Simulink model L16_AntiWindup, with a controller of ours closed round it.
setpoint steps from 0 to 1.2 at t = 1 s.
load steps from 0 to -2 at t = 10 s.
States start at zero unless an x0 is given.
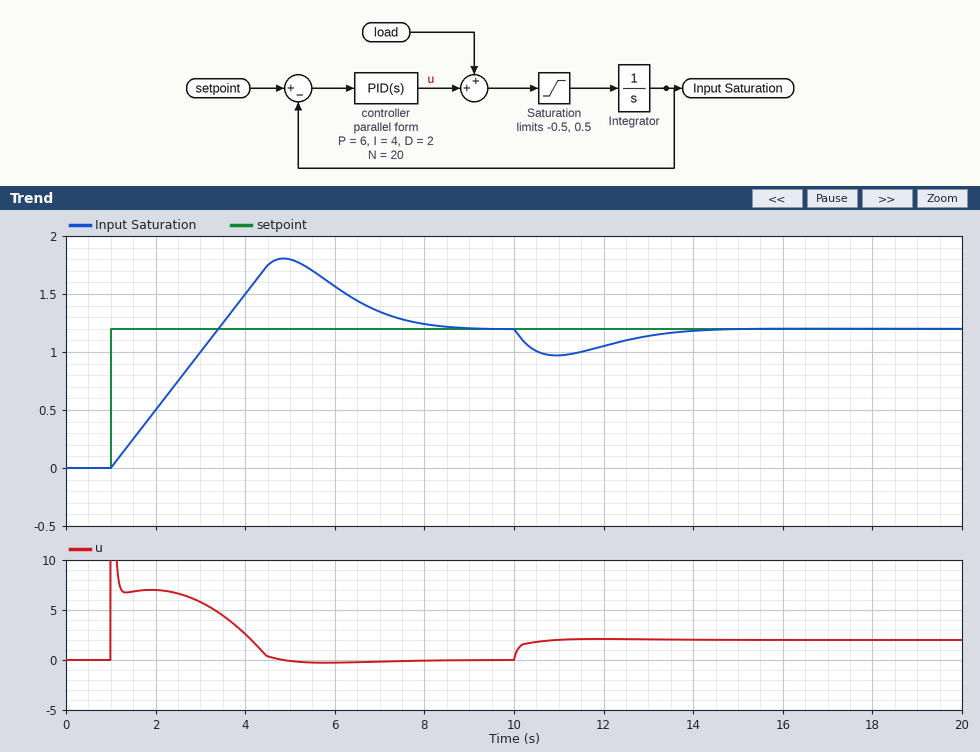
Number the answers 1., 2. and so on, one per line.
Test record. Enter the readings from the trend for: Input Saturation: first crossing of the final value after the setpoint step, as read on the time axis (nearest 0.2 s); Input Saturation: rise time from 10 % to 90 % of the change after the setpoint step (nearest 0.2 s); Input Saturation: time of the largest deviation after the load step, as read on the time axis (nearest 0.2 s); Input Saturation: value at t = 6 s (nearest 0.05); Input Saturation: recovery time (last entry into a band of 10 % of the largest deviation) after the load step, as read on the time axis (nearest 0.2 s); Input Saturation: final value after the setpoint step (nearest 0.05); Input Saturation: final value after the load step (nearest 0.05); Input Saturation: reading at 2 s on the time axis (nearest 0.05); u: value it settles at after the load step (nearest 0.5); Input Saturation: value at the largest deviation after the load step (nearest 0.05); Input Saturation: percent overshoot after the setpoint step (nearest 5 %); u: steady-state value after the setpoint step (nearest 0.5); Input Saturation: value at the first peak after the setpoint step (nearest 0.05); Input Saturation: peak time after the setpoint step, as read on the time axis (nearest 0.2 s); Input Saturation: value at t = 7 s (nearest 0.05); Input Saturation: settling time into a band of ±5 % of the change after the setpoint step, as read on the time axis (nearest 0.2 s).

1. 3.4 s
2. 2.0 s
3. 11.0 s
4. 1.55
5. 13.8 s
6. 1.20
7. 1.20
8. 0.50
9. 2.0
10. 0.95
11. 50 %
12. 0.0
13. 1.80
14. 4.8 s
15. 1.35
16. 7.8 s
